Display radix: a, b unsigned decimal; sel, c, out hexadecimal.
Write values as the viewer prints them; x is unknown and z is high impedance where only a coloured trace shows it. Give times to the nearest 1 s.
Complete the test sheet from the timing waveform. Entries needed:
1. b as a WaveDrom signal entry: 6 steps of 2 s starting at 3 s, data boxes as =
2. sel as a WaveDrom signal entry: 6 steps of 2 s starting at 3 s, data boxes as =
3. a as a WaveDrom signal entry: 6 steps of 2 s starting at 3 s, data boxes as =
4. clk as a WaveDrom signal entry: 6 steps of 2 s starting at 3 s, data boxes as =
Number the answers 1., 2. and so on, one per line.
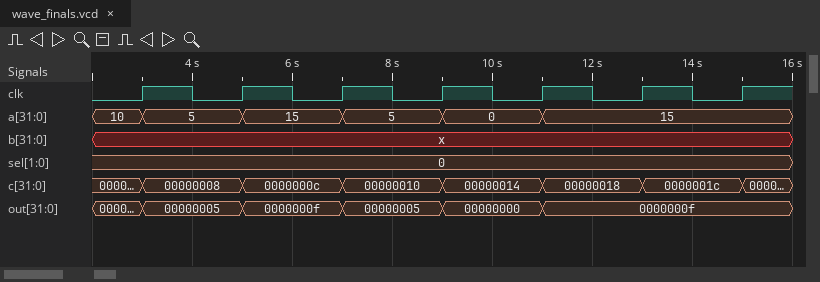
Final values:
1. {name: 'b', wave: 'x.....'}
2. {name: 'sel', wave: '=.....', data: '0'}
3. {name: 'a', wave: '=====.', data: '5 15 5 0 15'}
4. {name: 'clk', wave: 'p.....'}
